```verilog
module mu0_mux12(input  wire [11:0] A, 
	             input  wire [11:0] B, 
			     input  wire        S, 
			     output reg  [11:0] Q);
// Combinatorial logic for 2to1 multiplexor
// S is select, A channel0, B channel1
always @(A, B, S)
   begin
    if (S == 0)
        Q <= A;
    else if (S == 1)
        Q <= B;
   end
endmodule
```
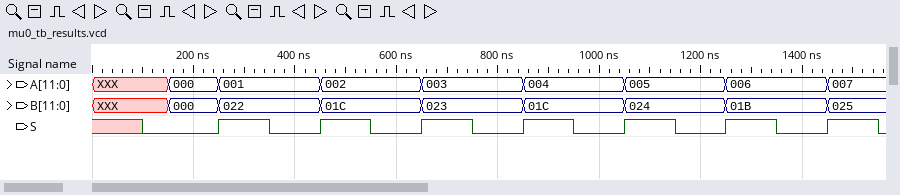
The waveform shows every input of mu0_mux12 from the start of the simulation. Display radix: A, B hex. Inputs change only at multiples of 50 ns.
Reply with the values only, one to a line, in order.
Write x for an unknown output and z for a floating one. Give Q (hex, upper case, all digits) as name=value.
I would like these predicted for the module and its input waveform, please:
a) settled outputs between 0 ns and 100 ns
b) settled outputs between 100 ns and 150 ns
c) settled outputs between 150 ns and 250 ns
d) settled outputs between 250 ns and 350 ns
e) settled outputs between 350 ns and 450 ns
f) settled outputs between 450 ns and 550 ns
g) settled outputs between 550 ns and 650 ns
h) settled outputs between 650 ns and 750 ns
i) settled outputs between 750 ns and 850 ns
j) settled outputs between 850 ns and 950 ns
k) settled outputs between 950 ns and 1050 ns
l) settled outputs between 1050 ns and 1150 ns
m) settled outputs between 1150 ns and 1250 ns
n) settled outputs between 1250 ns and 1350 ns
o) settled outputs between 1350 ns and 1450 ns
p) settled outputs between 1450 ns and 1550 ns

Q=x
Q=x
Q=000
Q=022
Q=001
Q=01C
Q=002
Q=023
Q=003
Q=01C
Q=004
Q=024
Q=005
Q=01B
Q=006
Q=025
